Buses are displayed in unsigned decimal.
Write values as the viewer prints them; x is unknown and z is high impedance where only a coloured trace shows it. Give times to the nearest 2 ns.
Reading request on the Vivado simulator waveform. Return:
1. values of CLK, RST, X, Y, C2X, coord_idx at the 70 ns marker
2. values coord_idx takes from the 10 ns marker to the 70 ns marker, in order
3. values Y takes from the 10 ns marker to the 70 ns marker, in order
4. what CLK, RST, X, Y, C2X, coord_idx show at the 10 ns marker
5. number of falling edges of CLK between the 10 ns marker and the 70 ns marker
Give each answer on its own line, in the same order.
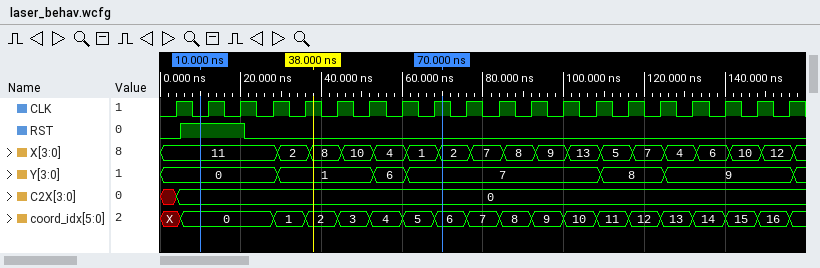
CLK=1, RST=0, X=2, Y=7, C2X=0, coord_idx=6
0, 1, 2, 3, 4, 5, 6
0, 1, 6, 7
CLK=0, RST=1, X=11, Y=0, C2X=0, coord_idx=0
7
